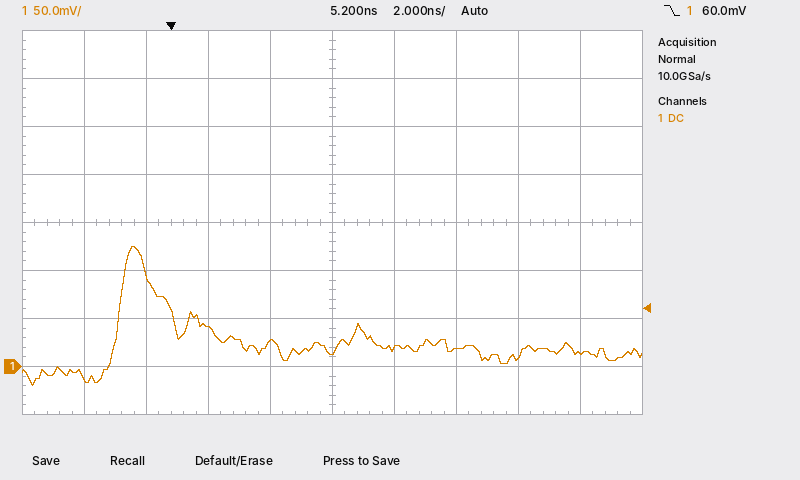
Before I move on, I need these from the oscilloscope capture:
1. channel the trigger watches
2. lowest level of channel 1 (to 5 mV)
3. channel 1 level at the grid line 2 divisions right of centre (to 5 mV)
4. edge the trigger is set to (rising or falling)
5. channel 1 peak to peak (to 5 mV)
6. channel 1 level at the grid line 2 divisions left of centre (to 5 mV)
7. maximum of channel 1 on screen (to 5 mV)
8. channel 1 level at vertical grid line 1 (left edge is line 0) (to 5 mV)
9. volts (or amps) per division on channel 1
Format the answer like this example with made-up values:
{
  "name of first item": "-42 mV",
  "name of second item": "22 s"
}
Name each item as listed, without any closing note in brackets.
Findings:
{
  "channel the trigger watches": "channel 1",
  "lowest level of channel 1": "-20 mV",
  "channel 1 level at the grid line 2 divisions right of centre": "20 mV",
  "edge the trigger is set to": "falling",
  "channel 1 peak to peak": "145 mV",
  "channel 1 level at the grid line 2 divisions left of centre": "40 mV",
  "maximum of channel 1 on screen": "125 mV",
  "channel 1 level at vertical grid line 1 (left edge is line 0)": "-10 mV",
  "volts (or amps) per division on channel 1": "50 mV"
}
